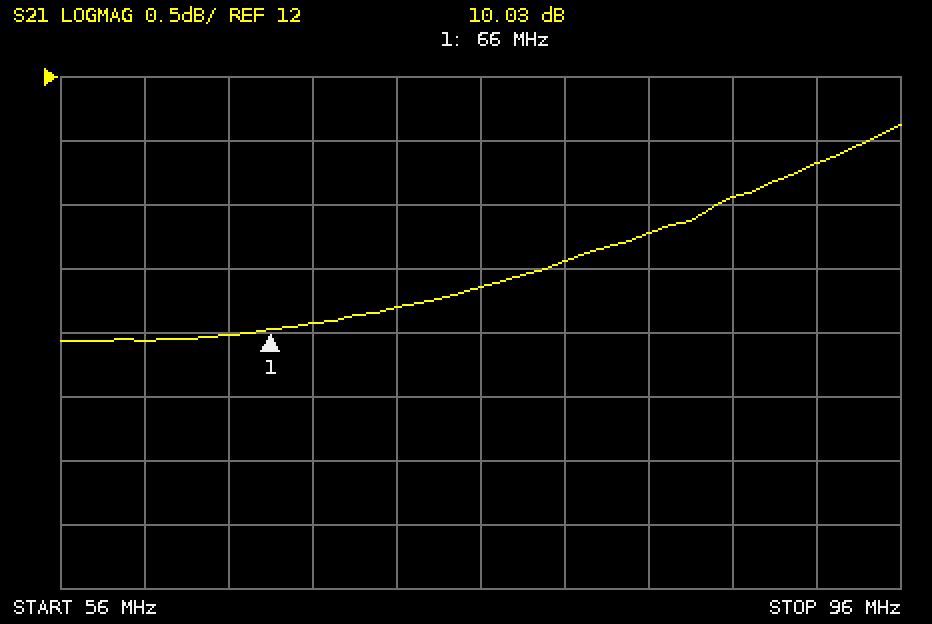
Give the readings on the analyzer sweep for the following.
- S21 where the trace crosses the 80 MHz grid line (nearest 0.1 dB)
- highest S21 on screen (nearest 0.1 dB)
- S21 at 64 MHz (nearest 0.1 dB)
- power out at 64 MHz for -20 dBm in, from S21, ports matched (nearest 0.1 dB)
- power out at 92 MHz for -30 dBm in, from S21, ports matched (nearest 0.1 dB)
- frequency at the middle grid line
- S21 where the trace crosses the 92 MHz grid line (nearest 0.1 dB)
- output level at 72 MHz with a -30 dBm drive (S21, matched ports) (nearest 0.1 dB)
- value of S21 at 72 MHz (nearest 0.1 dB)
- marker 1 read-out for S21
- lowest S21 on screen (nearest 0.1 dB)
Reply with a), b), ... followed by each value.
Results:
a) 10.6 dB
b) 11.6 dB
c) 10.0 dB
d) -10.0 dBm
e) -18.7 dBm
f) 76 MHz
g) 11.3 dB
h) -19.8 dBm
i) 10.2 dB
j) 10.03 dB
k) 9.9 dB
